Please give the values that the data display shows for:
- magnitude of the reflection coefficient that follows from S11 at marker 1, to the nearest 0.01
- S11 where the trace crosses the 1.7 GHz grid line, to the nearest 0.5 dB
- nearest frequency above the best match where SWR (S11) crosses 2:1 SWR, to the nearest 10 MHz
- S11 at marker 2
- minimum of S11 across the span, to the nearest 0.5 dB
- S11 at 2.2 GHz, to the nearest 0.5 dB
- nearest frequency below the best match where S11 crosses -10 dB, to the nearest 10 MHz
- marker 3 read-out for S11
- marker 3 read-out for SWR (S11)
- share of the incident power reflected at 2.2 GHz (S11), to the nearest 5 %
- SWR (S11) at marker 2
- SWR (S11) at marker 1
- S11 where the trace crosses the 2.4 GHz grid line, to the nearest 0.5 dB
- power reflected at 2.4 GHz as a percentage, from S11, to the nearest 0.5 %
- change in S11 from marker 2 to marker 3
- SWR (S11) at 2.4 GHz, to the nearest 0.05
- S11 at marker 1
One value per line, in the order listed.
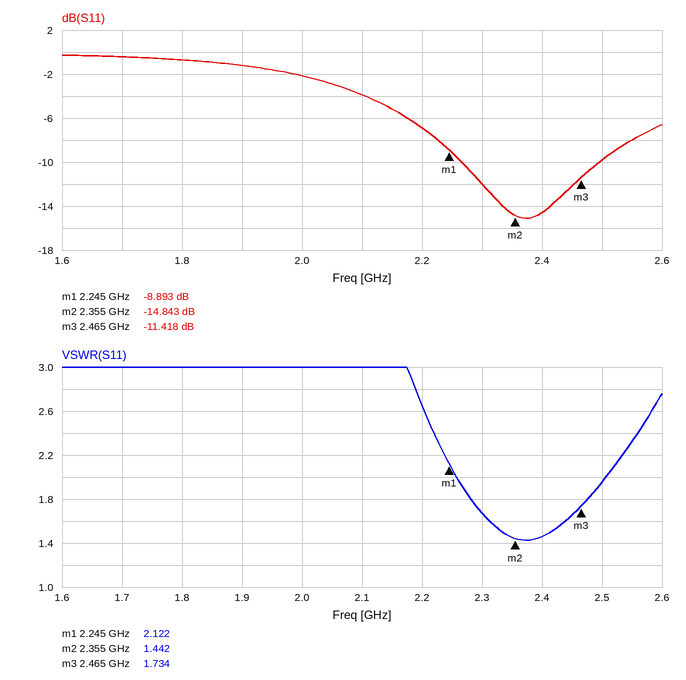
0.36
-0.5 dB
2.51 GHz
-14.843 dB
-15.0 dB
-7.0 dB
2.27 GHz
-11.418 dB
1.734
20 %
1.442
2.122
-14.5 dB
3.5 %
3.425 dB
1.45
-8.893 dB
